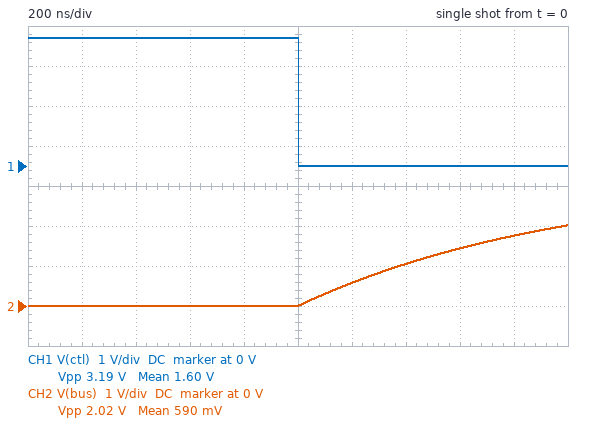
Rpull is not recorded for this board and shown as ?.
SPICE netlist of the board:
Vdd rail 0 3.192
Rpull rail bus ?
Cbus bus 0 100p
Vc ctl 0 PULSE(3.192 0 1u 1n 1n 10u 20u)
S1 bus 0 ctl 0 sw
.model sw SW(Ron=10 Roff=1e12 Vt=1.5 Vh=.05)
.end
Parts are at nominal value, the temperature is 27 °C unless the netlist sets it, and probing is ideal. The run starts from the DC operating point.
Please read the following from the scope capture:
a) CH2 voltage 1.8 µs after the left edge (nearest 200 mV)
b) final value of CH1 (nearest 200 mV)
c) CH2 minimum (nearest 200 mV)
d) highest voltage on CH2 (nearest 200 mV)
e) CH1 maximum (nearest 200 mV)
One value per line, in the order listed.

1.8 V
0 V
0 V
2.0 V
3.2 V
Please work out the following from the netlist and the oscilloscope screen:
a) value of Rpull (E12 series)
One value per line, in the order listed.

10 kΩ
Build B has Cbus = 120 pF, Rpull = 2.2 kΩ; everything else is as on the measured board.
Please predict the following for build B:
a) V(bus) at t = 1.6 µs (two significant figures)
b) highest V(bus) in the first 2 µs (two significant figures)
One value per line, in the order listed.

2.9 V
3.1 V
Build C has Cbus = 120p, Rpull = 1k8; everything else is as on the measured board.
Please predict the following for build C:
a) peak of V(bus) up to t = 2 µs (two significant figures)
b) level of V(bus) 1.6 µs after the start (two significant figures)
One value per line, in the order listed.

3.2 V
3.0 V
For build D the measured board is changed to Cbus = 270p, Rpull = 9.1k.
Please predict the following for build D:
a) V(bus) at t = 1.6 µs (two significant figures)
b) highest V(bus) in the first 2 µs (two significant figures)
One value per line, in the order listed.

690 mV
1.1 V
